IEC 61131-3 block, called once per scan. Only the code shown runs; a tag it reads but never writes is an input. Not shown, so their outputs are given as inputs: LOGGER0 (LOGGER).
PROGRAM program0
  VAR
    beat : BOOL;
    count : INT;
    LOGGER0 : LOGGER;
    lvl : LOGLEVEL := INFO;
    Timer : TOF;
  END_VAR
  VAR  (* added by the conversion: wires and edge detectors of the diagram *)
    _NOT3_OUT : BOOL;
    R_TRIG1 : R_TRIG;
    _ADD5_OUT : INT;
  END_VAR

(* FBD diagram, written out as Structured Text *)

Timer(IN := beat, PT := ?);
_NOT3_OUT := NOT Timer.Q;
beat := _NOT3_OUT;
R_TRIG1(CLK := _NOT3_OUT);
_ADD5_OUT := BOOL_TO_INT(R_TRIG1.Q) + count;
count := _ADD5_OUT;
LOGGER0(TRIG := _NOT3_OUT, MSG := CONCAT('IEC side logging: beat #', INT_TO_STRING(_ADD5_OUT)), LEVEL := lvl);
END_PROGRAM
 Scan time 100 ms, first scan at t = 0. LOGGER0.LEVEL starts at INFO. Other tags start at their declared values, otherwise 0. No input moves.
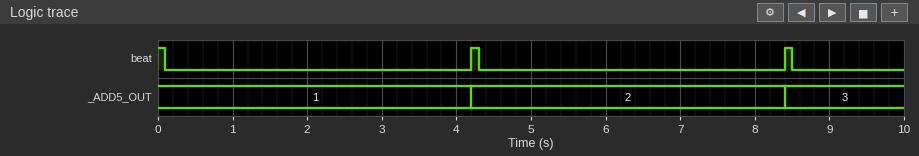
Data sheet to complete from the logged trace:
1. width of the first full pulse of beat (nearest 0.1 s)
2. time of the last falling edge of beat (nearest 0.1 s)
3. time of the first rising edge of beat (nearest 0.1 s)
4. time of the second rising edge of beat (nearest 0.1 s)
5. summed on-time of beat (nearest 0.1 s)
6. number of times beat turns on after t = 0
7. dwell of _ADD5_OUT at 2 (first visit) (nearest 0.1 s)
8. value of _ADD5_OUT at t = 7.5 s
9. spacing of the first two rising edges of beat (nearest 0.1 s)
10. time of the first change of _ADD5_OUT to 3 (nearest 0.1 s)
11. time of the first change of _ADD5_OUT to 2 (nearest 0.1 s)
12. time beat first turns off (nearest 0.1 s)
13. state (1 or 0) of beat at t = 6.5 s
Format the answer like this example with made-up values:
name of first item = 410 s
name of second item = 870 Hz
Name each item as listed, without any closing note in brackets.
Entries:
width of the first full pulse of beat = 0.1 s
time of the last falling edge of beat = 8.5 s
time of the first rising edge of beat = 4.2 s
time of the second rising edge of beat = 8.4 s
summed on-time of beat = 0.3 s
number of times beat turns on after t = 0 = 2
dwell of _ADD5_OUT at 2 (first visit) = 4.2 s
value of _ADD5_OUT at t = 7.5 s = 2
spacing of the first two rising edges of beat = 4.2 s
time of the first change of _ADD5_OUT to 3 = 8.4 s
time of the first change of _ADD5_OUT to 2 = 4.2 s
time beat first turns off = 0.1 s
state (1 or 0) of beat at t = 6.5 s = 0
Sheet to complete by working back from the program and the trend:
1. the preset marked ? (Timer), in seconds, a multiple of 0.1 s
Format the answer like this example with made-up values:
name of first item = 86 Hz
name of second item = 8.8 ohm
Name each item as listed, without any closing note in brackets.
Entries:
the preset marked ? (Timer), in seconds, a multiple of 0.1 s = 4.0 s
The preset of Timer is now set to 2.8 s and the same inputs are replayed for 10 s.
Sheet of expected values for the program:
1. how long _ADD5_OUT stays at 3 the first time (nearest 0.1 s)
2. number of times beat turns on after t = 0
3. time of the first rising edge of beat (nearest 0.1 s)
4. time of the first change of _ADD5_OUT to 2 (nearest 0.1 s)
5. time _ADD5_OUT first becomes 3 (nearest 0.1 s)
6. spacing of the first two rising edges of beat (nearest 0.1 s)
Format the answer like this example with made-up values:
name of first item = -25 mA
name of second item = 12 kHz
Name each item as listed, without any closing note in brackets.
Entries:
how long _ADD5_OUT stays at 3 the first time = 3.0 s
number of times beat turns on after t = 0 = 3
time of the first rising edge of beat = 3.0 s
time of the first change of _ADD5_OUT to 2 = 3.0 s
time _ADD5_OUT first becomes 3 = 6.0 s
spacing of the first two rising edges of beat = 3.0 s
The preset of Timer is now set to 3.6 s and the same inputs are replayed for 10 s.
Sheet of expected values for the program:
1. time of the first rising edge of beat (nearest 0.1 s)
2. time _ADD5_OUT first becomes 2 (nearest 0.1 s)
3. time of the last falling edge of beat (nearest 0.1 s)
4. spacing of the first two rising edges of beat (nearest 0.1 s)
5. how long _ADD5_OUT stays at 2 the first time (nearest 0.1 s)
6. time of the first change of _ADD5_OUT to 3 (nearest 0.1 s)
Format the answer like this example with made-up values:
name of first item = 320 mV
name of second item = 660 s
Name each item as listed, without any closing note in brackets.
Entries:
time of the first rising edge of beat = 3.8 s
time _ADD5_OUT first becomes 2 = 3.8 s
time of the last falling edge of beat = 7.7 s
spacing of the first two rising edges of beat = 3.8 s
how long _ADD5_OUT stays at 2 the first time = 3.8 s
time of the first change of _ADD5_OUT to 3 = 7.6 s
